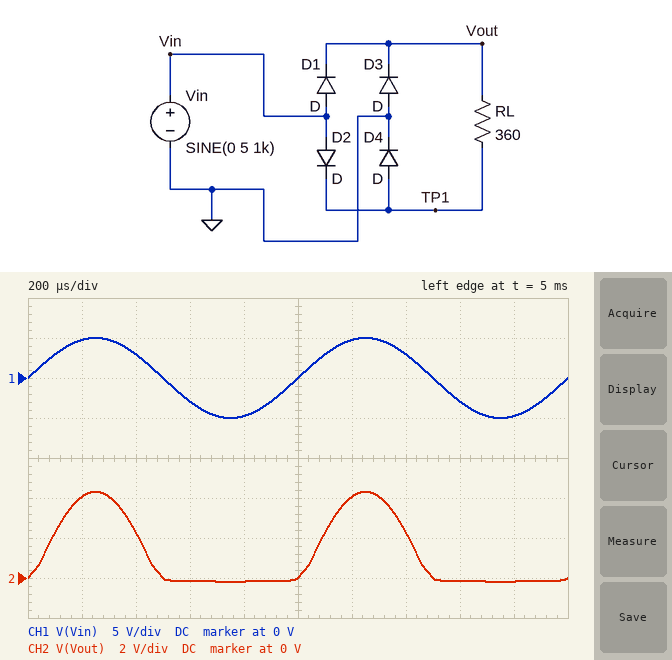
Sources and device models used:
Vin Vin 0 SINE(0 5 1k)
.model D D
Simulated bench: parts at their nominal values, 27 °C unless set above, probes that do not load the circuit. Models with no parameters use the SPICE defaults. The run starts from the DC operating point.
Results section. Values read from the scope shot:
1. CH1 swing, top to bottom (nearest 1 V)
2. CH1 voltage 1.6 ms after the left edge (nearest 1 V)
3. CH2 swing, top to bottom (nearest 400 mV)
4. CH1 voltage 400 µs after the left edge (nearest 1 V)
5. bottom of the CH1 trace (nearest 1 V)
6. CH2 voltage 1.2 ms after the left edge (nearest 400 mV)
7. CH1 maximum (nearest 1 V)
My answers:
10 V
-3 V
4.4 V
3 V
-5 V
4.0 V
5 V
